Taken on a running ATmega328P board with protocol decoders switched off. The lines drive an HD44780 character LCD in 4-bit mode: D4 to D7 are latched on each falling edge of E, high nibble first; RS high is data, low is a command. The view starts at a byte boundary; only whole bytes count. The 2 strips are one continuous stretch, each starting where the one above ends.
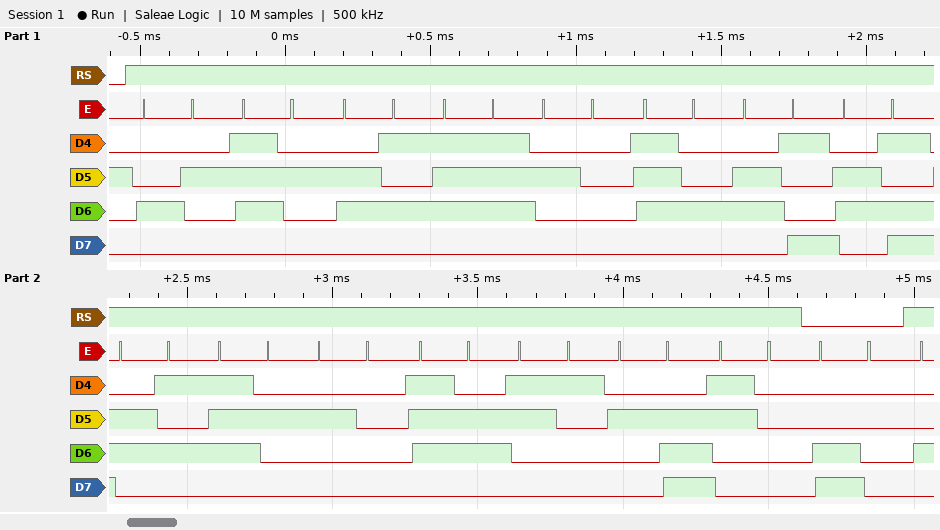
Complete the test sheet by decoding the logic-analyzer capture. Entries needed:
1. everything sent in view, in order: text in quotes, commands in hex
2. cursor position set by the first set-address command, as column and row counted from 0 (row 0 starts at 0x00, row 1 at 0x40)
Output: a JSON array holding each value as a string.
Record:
["\"Brew timer v1.0\" 0xC0", "column 0, row 1"]
